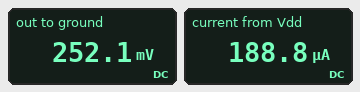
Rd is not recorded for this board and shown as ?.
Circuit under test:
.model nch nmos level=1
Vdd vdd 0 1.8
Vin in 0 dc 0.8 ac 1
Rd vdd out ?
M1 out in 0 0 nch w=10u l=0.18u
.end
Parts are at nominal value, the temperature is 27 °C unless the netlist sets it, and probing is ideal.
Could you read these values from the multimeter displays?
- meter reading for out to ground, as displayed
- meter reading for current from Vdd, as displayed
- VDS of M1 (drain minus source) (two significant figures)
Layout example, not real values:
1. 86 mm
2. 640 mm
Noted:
1. 252.1 mV
2. 188.8 µA
3. 250 mV
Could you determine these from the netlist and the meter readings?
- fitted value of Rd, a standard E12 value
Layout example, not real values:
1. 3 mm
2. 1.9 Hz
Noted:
1. 8.2 kΩ
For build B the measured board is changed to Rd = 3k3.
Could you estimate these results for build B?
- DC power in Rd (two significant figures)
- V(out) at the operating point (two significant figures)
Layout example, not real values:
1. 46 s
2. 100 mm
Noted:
1. 390 µW
2. 660 mV
